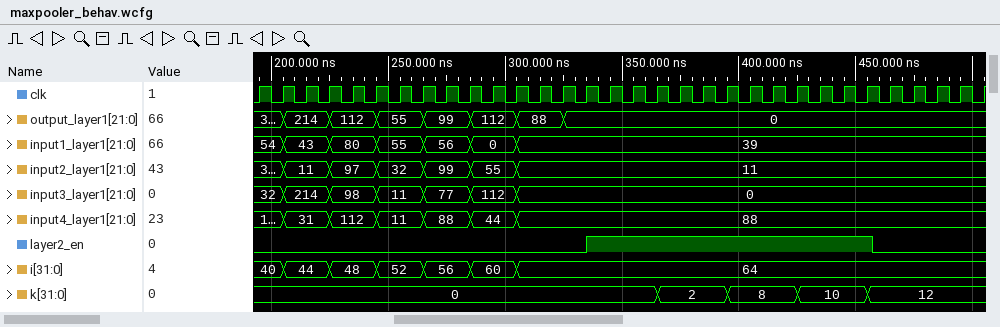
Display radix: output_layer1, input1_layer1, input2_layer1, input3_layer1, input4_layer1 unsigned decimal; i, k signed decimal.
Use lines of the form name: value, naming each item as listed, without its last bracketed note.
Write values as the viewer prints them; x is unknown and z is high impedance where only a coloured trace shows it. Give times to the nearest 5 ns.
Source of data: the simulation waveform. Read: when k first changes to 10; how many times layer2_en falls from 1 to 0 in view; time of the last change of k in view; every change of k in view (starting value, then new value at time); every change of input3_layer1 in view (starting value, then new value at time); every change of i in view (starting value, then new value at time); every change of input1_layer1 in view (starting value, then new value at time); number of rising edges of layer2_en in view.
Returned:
when k first changes to 10: 425 ns
how many times layer2_en falls from 1 to 0 in view: 1
time of the last change of k in view: 455 ns
every change of k in view: 0, 2 at 365 ns, 8 at 395 ns, 10 at 425 ns, 12 at 455 ns
every change of input3_layer1 in view: 32, 214 at 205 ns, 98 at 225 ns, 11 at 245 ns, 77 at 265 ns, 112 at 285 ns, 0 at 305 ns
every change of i in view: 40, 44 at 205 ns, 48 at 225 ns, 52 at 245 ns, 56 at 265 ns, 60 at 285 ns, 64 at 305 ns
every change of input1_layer1 in view: 54, 43 at 205 ns, 80 at 225 ns, 55 at 245 ns, 56 at 265 ns, 0 at 285 ns, 39 at 305 ns
number of rising edges of layer2_en in view: 1
